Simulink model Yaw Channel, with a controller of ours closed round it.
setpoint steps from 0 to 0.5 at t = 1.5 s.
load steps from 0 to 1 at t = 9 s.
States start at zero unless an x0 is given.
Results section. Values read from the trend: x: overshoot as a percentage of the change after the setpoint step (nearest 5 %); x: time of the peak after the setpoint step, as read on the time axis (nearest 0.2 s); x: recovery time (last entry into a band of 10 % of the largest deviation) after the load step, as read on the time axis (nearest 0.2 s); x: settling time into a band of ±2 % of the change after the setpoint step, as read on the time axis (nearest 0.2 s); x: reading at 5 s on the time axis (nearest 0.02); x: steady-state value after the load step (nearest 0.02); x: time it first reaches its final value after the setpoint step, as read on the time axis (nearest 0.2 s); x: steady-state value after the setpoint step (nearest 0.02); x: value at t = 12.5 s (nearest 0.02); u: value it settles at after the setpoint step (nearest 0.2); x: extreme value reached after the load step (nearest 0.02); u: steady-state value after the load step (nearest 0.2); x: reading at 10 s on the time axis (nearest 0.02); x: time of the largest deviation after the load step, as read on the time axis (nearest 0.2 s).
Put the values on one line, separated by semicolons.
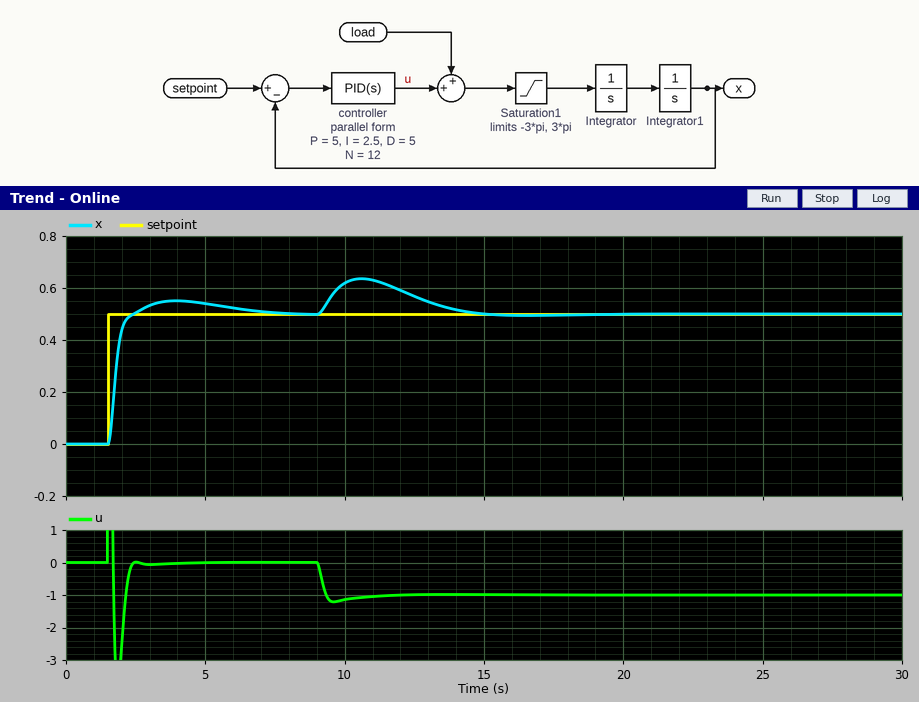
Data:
10 %; 4.0 s; 14.2 s; 7.0 s; 0.54; 0.50; 2.4 s; 0.50; 0.56; 0.0; 0.64; -1.0; 0.62; 10.6 s
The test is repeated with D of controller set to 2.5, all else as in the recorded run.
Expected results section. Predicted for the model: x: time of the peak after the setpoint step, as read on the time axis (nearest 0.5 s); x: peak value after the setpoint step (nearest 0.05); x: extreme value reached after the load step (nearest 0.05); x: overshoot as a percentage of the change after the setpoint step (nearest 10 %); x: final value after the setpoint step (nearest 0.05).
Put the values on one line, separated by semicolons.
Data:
2.5 s; 0.70; 0.70; 40 %; 0.50
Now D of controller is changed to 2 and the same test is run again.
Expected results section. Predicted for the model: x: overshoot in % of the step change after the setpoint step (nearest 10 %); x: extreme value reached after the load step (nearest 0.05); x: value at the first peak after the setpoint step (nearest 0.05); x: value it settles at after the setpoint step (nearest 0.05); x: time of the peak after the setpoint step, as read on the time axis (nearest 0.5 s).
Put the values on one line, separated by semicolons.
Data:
50 %; 0.70; 0.75; 0.50; 2.5 s
